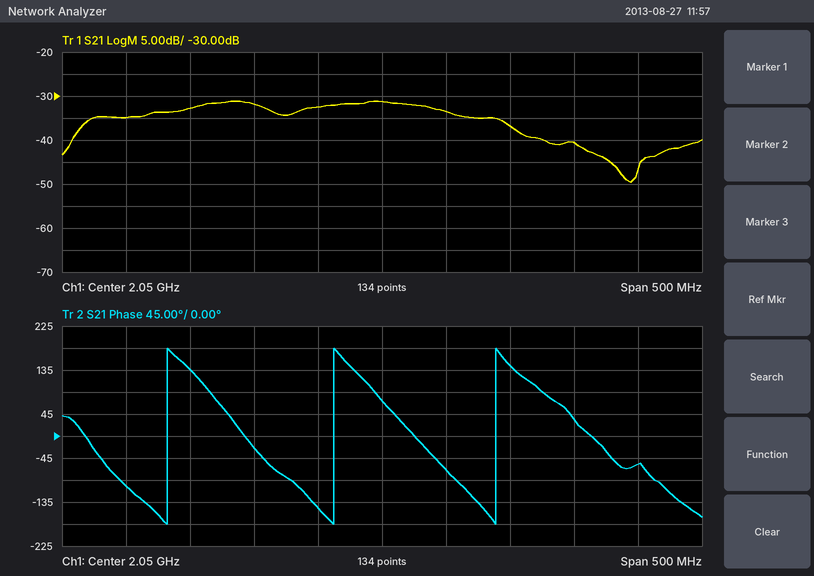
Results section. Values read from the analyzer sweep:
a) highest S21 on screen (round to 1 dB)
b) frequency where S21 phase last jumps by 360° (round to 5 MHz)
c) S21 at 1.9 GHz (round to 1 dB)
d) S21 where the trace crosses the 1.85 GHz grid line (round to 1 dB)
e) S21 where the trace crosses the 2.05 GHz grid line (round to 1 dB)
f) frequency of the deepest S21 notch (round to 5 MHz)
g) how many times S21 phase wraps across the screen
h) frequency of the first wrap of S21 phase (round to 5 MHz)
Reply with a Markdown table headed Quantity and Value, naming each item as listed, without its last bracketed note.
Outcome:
| Quantity | Value |
|---|---|
| highest S21 on screen | -31 dB |
| frequency where S21 phase last jumps by 360° | 2.140 GHz |
| S21 at 1.9 GHz | -33 dB |
| S21 where the trace crosses the 1.85 GHz grid line | -35 dB |
| S21 where the trace crosses the 2.05 GHz grid line | -31 dB |
| frequency of the deepest S21 notch | 2.245 GHz |
| how many times S21 phase wraps across the screen | 3 |
| frequency of the first wrap of S21 phase | 1.880 GHz |
